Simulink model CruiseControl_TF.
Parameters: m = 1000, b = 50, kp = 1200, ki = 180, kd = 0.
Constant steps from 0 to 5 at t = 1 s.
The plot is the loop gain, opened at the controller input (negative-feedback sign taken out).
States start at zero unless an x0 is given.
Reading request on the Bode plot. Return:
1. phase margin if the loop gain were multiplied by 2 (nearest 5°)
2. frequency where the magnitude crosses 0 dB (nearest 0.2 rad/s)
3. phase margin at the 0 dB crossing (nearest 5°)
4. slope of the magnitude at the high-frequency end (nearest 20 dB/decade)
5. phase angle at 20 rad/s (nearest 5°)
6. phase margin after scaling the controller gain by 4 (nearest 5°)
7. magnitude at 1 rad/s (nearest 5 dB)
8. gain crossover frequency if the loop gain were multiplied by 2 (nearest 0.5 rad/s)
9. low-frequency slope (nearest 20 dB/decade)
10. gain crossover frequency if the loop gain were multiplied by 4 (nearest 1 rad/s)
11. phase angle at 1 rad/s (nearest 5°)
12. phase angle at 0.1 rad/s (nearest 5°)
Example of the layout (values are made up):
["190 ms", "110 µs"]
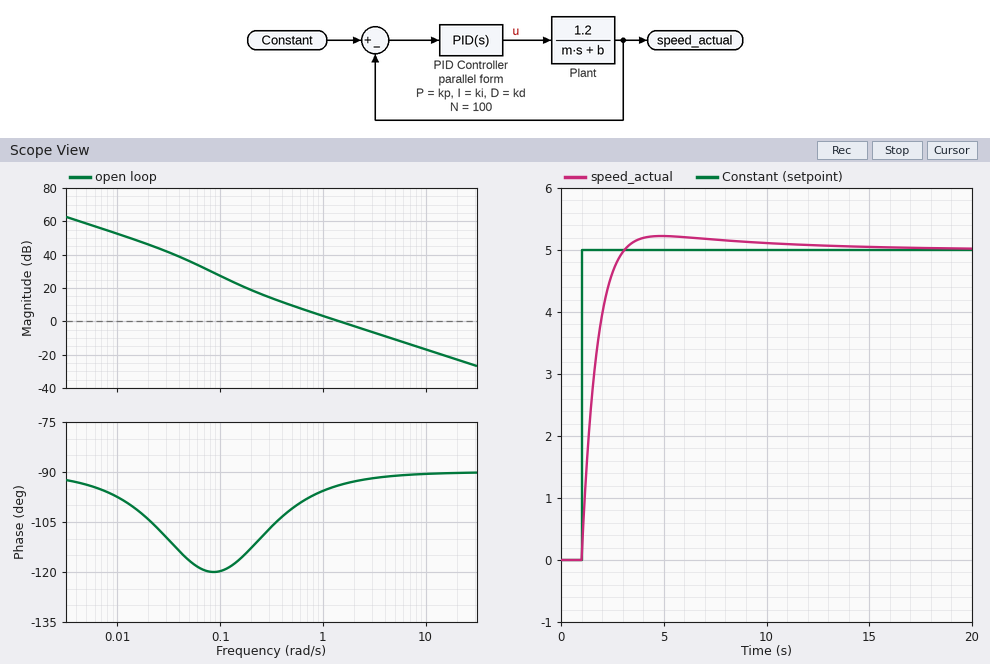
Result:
["90°", "1.4 rad/s", "85°", "-20 dB/decade", "-90°", "90°", "5 dB", "3.0 rad/s", "-20 dB/decade", "6 rad/s", "-95°", "-120°"]
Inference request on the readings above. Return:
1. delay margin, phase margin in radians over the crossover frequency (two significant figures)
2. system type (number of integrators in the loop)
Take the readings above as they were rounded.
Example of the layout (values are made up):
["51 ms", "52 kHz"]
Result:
["1.1 s", "1"]
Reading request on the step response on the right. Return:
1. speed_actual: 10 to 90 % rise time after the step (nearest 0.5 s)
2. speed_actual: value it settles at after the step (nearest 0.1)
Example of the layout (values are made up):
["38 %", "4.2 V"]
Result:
["1.5 s", "5.0"]
